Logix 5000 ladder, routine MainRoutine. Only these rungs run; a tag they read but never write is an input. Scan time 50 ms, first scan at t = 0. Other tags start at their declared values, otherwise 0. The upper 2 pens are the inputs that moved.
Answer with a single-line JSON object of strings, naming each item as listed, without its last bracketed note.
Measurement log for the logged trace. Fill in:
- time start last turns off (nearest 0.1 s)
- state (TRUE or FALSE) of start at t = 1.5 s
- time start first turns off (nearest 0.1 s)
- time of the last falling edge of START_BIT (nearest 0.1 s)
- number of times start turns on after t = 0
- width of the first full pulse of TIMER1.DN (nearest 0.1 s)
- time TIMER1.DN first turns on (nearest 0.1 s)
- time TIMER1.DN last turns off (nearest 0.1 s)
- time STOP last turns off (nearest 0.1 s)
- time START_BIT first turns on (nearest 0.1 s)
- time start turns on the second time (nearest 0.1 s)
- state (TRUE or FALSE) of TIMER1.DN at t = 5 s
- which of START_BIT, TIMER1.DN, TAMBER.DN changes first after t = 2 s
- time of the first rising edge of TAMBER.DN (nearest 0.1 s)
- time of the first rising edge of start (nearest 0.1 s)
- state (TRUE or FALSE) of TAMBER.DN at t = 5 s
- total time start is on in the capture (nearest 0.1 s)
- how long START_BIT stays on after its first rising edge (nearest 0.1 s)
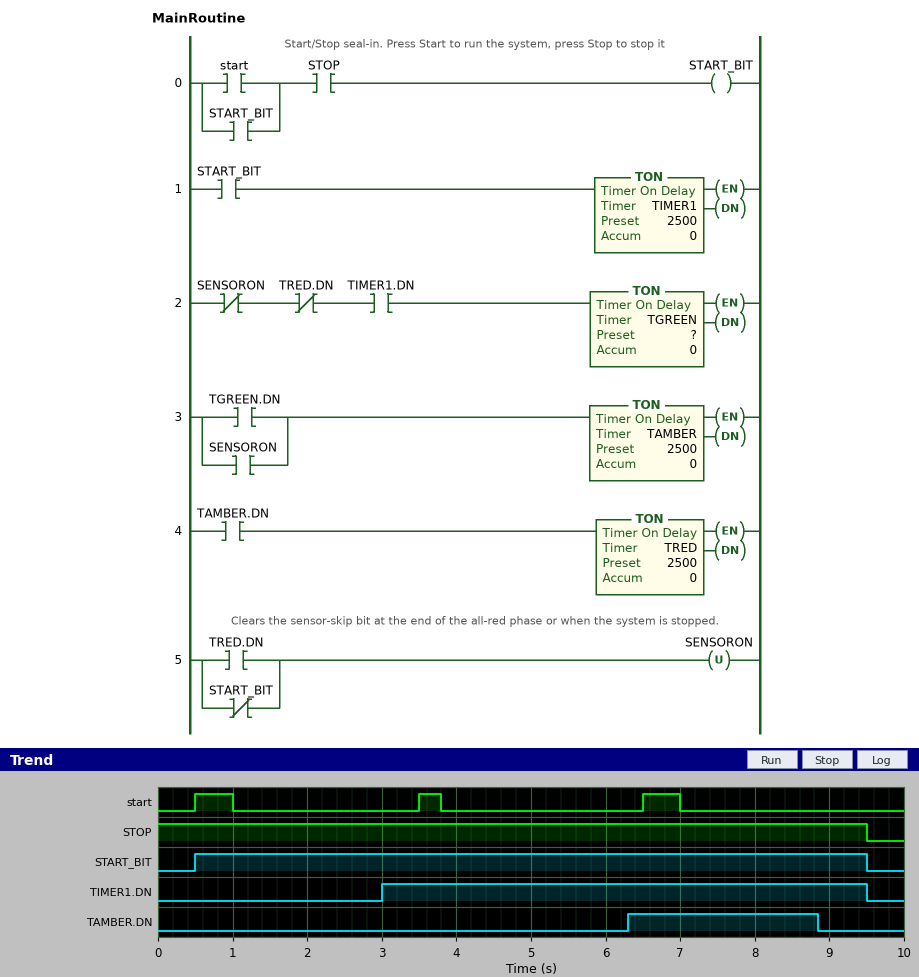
{"time start last turns off": "7.0 s", "state (TRUE or FALSE) of start at t = 1.5 s": "FALSE", "time start first turns off": "1.0 s", "time of the last falling edge of START_BIT": "9.5 s", "number of times start turns on after t = 0": "3", "width of the first full pulse of TIMER1.DN": "6.5 s", "time TIMER1.DN first turns on": "3.0 s", "time TIMER1.DN last turns off": "9.5 s", "time STOP last turns off": "9.5 s", "time START_BIT first turns on": "0.5 s", "time start turns on the second time": "3.5 s", "state (TRUE or FALSE) of TIMER1.DN at t = 5 s": "TRUE", "which of START_BIT, TIMER1.DN, TAMBER.DN changes first after t = 2 s": "TIMER1.DN", "time of the first rising edge of TAMBER.DN": "6.3 s", "time of the first rising edge of start": "0.5 s", "state (TRUE or FALSE) of TAMBER.DN at t = 5 s": "FALSE", "total time start is on in the capture": "1.3 s", "how long START_BIT stays on after its first rising edge": "9.0 s"}
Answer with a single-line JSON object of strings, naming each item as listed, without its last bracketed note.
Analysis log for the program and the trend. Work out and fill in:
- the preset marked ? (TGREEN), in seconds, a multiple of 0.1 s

{"the preset marked ? (TGREEN), in seconds, a multiple of 0.1 s": "0.8 s"}
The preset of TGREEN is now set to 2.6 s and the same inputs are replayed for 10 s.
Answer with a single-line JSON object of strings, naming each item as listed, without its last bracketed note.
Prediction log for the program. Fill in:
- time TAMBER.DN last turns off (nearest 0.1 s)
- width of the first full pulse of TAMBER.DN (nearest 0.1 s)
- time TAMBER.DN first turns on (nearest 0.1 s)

{"time TAMBER.DN last turns off": "9.5 s", "width of the first full pulse of TAMBER.DN": "1.4 s", "time TAMBER.DN first turns on": "8.1 s"}
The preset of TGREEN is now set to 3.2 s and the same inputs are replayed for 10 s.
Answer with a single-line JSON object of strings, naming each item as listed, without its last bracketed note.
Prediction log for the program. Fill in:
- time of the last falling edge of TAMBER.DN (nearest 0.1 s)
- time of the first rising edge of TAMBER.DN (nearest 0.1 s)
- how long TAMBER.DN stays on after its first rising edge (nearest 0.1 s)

{"time of the last falling edge of TAMBER.DN": "9.5 s", "time of the first rising edge of TAMBER.DN": "8.7 s", "how long TAMBER.DN stays on after its first rising edge": "0.8 s"}
